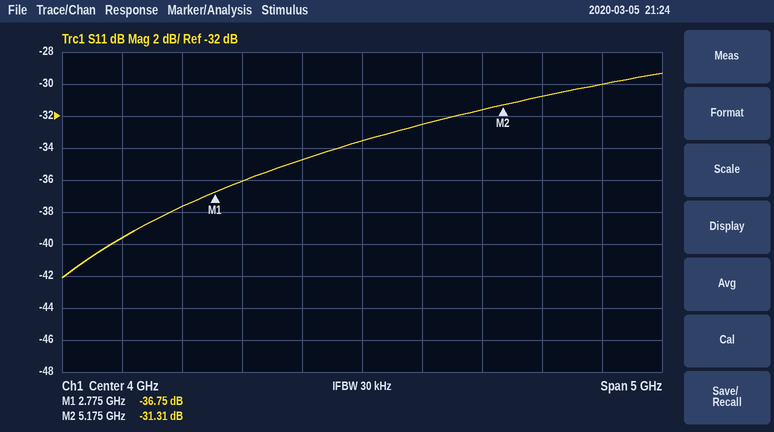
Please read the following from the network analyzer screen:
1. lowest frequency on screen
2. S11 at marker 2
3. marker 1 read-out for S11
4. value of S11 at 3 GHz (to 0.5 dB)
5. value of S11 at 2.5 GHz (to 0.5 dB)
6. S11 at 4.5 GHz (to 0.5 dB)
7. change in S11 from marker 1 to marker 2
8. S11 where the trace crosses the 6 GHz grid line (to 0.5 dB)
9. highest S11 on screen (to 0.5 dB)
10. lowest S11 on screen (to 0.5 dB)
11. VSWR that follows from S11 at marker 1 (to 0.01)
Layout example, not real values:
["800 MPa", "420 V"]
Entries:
["1.5 GHz", "-31.31 dB", "-36.75 dB", "-36.0 dB", "-37.5 dB", "-32.5 dB", "5.44 dB", "-30.0 dB", "-29.5 dB", "-42.0 dB", "1.03"]
